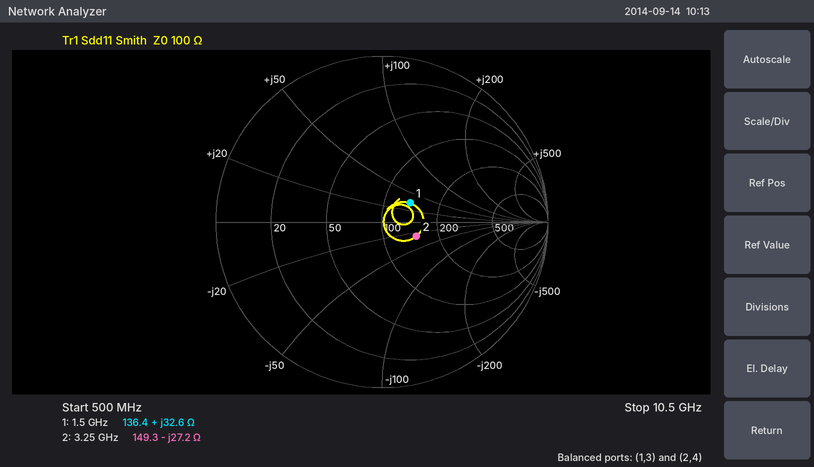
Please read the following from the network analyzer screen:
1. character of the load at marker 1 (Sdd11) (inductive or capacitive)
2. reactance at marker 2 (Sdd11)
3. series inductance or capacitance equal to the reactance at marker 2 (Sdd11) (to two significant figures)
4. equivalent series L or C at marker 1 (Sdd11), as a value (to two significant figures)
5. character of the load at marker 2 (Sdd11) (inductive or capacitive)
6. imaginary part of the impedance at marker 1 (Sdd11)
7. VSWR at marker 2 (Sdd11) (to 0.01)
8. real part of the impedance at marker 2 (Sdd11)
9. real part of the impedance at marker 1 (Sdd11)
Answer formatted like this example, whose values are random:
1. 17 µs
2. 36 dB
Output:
1. inductive
2. -27.2 Ω
3. 1.8 pF
4. 3.5 nH
5. capacitive
6. +32.6 Ω
7. 1.58
8. 149.3 Ω
9. 136.4 Ω
